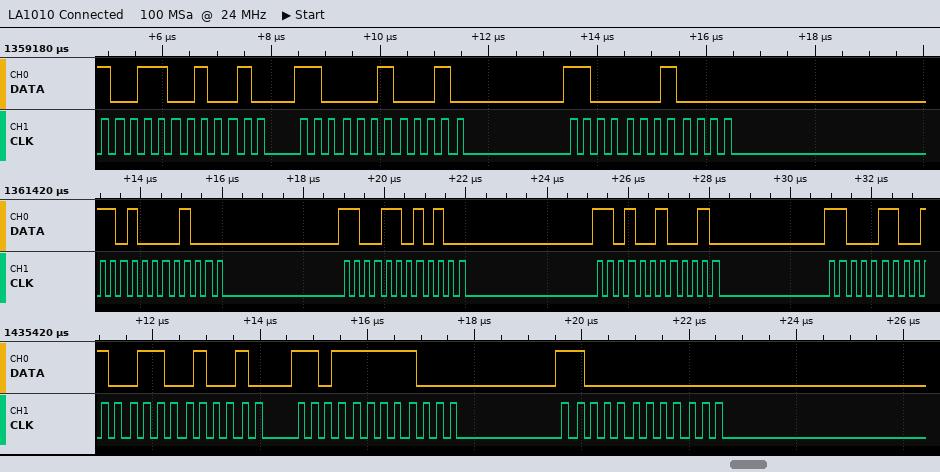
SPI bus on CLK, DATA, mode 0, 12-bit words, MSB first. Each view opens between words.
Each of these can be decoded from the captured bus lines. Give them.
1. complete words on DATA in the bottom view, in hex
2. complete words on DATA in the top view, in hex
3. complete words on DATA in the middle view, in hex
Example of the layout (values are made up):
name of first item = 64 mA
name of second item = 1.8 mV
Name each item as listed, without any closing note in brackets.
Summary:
complete words on DATA in the bottom view, in hex = 992, DF8, C00
complete words on DATA in the top view, in hex = 992, C22, C10
complete words on DATA in the middle view, in hex = D08, CD4, D22
